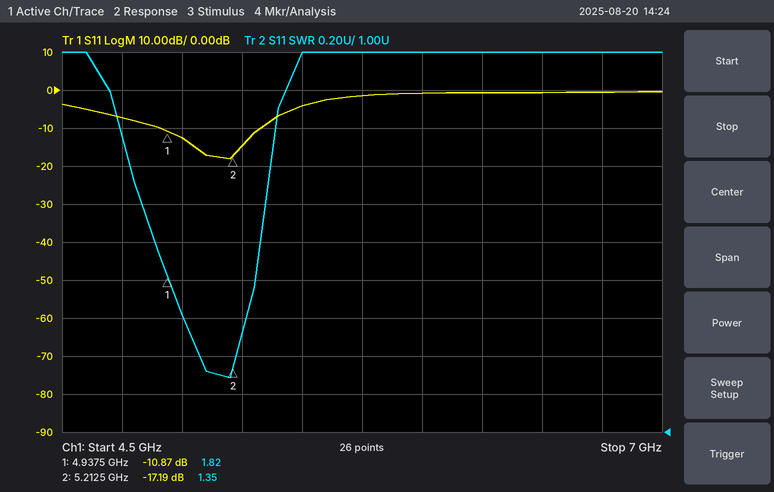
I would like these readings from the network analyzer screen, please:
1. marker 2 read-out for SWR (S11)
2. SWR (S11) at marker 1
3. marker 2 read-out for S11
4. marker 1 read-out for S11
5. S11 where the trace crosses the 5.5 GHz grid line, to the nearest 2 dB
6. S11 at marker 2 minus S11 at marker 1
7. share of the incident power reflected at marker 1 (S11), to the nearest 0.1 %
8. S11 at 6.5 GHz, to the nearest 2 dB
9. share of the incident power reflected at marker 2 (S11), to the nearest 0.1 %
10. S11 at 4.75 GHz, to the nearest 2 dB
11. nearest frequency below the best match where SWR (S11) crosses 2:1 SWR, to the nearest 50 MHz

1.35
1.82
-17.19 dB
-10.87 dB
-4 dB
-6.32 dB
8.2 %
0 dB
1.9 %
-8 dB
4.90 GHz
